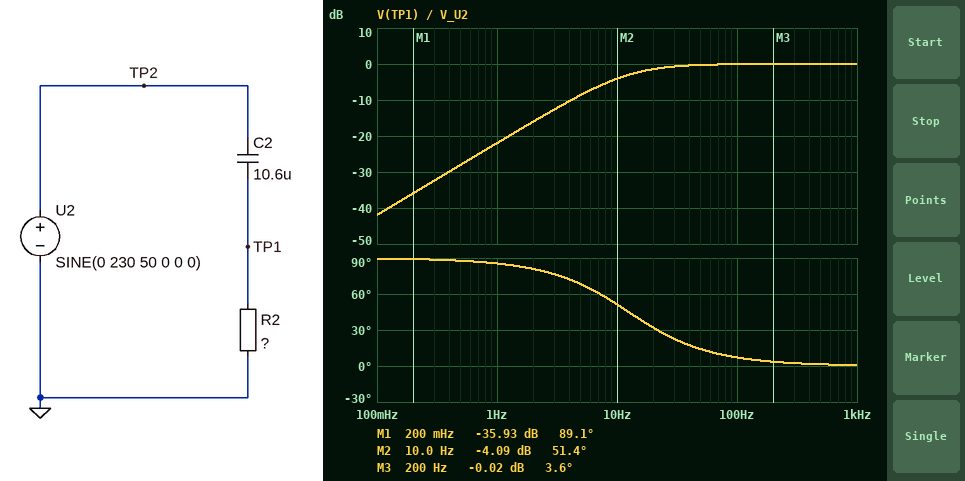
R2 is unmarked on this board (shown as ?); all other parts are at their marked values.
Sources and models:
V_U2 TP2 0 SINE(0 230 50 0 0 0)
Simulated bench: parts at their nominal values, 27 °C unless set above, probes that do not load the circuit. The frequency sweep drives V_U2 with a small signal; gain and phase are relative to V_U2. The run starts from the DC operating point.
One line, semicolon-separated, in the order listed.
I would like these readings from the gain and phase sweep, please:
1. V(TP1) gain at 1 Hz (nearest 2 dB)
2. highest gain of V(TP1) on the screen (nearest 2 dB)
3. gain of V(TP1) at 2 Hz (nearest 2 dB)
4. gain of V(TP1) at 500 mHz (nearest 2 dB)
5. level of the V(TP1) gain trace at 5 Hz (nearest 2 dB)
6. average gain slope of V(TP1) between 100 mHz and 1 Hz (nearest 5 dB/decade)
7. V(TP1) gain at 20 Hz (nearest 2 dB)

-22 dB; 0 dB; -16 dB; -28 dB; -8 dB; 20 dB/decade; -2 dB
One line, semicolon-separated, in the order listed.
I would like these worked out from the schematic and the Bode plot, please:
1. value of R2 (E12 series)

1.2 kΩ
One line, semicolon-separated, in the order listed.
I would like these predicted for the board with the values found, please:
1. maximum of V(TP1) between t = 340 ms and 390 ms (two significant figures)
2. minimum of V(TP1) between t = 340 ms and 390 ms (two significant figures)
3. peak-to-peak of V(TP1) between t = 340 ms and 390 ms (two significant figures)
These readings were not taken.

220 V; -220 V; 450 V
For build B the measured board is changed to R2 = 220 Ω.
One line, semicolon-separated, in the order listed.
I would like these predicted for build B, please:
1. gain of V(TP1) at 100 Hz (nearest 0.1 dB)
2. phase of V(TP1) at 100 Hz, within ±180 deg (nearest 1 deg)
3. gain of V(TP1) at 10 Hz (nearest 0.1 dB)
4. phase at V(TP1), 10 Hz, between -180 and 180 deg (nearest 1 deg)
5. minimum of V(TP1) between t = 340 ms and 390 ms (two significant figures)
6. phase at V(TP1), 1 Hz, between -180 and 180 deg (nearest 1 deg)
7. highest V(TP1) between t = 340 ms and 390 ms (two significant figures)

-1.7 dB; 34 deg; -16.8 dB; 82 deg; -140 V; 89 deg; 140 V
